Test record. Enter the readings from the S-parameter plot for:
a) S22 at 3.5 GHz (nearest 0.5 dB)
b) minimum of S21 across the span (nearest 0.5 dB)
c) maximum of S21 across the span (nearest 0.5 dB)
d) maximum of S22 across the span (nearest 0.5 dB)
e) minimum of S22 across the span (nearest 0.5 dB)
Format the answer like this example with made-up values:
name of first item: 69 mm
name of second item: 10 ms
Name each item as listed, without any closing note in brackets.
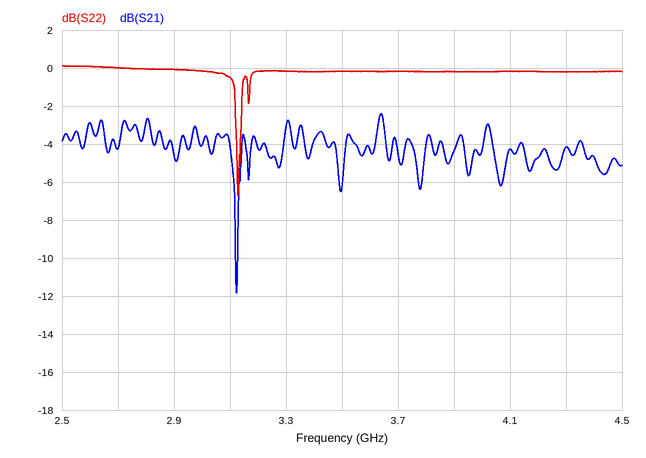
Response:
S22 at 3.5 GHz: 0.0 dB
minimum of S21 across the span: -12.0 dB
maximum of S21 across the span: -2.5 dB
maximum of S22 across the span: 0.0 dB
minimum of S22 across the span: -6.5 dB
